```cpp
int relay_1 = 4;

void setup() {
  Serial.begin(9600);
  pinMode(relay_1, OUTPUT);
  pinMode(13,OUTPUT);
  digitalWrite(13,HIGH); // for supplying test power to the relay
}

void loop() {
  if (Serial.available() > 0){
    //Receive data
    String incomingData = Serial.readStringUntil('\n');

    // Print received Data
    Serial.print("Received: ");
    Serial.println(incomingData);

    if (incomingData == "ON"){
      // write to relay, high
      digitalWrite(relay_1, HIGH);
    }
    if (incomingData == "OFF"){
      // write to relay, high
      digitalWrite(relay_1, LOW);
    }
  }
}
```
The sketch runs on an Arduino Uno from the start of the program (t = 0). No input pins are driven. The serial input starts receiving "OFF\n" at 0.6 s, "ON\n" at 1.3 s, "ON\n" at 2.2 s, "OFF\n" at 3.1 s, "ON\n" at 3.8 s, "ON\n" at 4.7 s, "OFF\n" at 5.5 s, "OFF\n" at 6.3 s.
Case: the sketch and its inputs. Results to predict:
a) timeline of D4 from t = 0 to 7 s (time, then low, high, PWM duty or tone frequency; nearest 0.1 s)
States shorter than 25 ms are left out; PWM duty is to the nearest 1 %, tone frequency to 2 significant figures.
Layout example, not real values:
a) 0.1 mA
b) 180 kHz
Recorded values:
a) 0 s low; 1.3 s high; 3.1 s low; 3.8 s high; 5.5 s low
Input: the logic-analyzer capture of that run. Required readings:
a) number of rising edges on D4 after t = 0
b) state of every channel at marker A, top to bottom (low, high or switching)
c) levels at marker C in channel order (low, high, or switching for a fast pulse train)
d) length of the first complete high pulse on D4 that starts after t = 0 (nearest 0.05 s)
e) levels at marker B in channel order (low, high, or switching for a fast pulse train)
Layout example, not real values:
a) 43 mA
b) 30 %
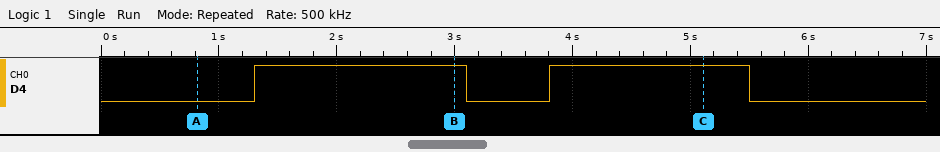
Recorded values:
a) 2
b) D4 low
c) D4 high
d) 1.80 s
e) D4 high
